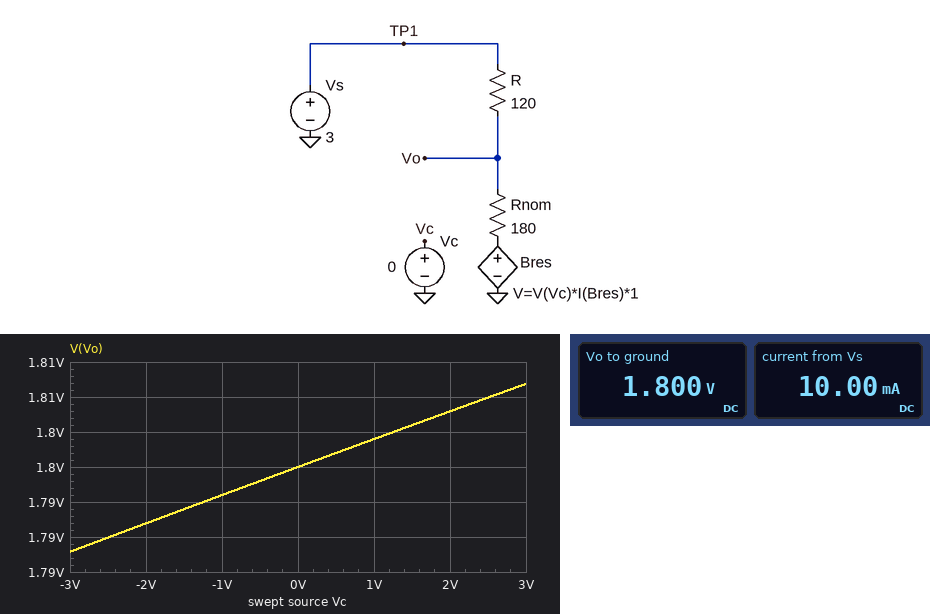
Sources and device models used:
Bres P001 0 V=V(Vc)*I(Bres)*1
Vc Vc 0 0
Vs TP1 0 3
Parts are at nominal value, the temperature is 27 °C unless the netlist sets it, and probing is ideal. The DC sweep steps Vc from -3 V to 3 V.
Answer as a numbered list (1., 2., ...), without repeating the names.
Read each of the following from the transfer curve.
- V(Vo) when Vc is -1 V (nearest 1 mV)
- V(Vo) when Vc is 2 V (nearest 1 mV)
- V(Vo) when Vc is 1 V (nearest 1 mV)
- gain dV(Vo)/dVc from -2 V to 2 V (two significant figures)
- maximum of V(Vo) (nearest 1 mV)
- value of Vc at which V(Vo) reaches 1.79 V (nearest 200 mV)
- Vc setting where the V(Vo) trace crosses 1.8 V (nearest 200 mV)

1. 1.796 V
2. 1.808 V
3. 1.804 V
4. 0.0040 V/V
5. 1.812 V
6. -1.2 V
7. 1.2 V
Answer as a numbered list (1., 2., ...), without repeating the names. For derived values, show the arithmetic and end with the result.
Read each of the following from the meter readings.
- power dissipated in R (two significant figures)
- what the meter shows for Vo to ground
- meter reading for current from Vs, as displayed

1. (3 V - 1.8 V)^2 / 120 Ω = 12 mW
2. 1.800 V
3. 10.00 mA
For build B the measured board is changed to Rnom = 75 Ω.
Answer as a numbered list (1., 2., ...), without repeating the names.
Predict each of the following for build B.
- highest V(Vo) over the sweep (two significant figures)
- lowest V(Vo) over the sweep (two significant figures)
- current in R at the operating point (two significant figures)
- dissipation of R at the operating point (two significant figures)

1. 1.2 V
2. 1.1 V
3. 15 mA
4. 28 mW
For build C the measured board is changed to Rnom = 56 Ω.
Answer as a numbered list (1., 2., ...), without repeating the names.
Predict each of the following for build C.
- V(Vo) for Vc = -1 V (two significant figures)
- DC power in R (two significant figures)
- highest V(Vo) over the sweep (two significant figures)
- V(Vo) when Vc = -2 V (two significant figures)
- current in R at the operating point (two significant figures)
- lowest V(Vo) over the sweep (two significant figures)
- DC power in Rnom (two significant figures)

1. 940 mV
2. 35 mW
3. 990 mV
4. 930 mV
5. 17 mA
6. 920 mV
7. 16 mW
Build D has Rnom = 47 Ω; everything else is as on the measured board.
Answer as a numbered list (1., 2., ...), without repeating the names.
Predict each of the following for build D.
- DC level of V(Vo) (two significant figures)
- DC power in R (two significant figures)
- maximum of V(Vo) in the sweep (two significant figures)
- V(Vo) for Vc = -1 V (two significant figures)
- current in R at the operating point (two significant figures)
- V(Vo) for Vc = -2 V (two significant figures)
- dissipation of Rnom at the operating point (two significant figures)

1. 840 mV
2. 39 mW
3. 880 mV
4. 830 mV
5. 18 mA
6. 820 mV
7. 15 mW
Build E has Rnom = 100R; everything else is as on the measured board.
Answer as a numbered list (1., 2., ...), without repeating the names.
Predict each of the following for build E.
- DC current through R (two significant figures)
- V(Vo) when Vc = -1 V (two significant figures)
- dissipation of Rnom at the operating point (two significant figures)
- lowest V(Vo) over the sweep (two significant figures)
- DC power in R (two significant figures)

1. 14 mA
2. 1.4 V
3. 19 mW
4. 1.3 V
5. 22 mW
